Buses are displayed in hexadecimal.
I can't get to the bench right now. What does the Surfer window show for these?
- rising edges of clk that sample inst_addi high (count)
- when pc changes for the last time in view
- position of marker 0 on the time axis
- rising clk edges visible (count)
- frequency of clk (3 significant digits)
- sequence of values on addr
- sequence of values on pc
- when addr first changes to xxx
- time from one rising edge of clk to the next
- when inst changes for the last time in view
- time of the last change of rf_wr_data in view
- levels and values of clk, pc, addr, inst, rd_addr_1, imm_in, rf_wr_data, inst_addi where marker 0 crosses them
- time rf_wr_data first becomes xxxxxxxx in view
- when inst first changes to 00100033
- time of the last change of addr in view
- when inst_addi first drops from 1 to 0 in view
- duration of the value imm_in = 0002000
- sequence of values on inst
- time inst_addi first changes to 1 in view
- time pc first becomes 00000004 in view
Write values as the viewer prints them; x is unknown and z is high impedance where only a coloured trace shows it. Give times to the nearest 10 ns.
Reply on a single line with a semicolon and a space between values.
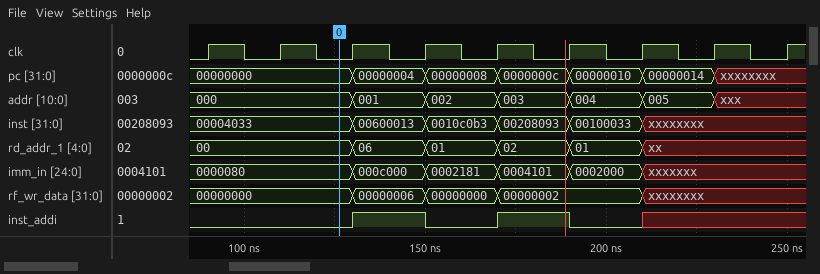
2; 230 ns; 130 ns; 9; 50.0 MHz; 000, 001, 002, 003, 004, 005, xxx; 00000000, 00000004, 00000008, 0000000c, 00000010, 00000014, xxxxxxxx; 230 ns; 20 ns; 210 ns; 210 ns; clk=0, pc=00000000, addr=000, inst=00004033, rd_addr_1=00, imm_in=0000080, rf_wr_data=00000000, inst_addi=0; 210 ns; 190 ns; 230 ns; 150 ns; 20 ns; 00004033, 00600013, 0010c0b3, 00208093, 00100033, xxxxxxxx; 130 ns; 130 ns
